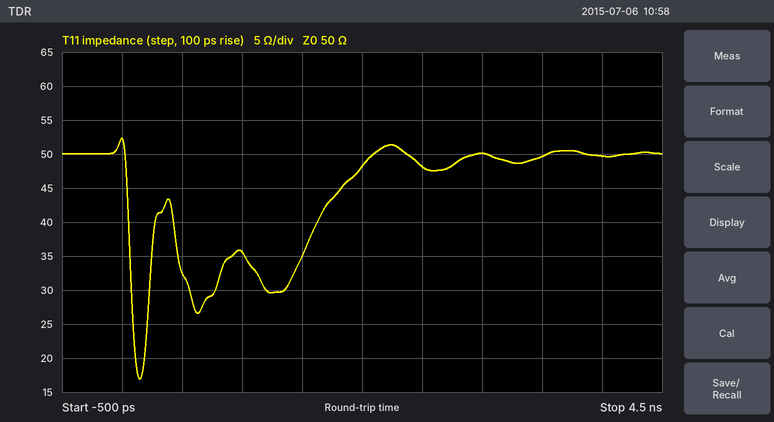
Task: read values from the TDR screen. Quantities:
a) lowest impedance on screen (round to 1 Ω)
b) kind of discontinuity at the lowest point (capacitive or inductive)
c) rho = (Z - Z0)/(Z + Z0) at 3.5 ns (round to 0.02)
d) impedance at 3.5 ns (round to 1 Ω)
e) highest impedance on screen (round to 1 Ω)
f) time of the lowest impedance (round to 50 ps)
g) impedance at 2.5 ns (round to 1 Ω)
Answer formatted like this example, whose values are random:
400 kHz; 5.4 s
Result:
17 Ω; capacitive; 0.00; 50 Ω; 52 Ω; 150 ps; 48 Ω
